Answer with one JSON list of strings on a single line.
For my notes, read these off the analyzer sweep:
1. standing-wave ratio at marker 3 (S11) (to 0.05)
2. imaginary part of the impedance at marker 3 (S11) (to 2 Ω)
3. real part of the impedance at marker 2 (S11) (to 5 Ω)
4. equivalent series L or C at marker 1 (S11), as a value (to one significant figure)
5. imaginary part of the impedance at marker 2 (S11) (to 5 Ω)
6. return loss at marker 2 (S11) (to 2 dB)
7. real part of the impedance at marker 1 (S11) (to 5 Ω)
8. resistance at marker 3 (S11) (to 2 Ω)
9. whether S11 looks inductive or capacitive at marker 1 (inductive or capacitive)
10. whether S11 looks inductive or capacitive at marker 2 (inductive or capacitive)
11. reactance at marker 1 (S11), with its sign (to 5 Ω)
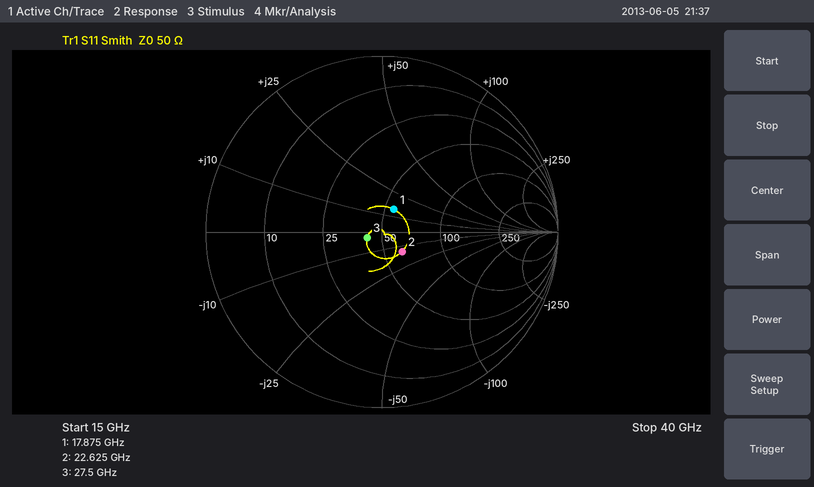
["1.20", "-2 Ω", "60 Ω", "100 pH", "-15 Ω", "16 dB", "55 Ω", "42 Ω", "inductive", "capacitive", "+15 Ω"]
